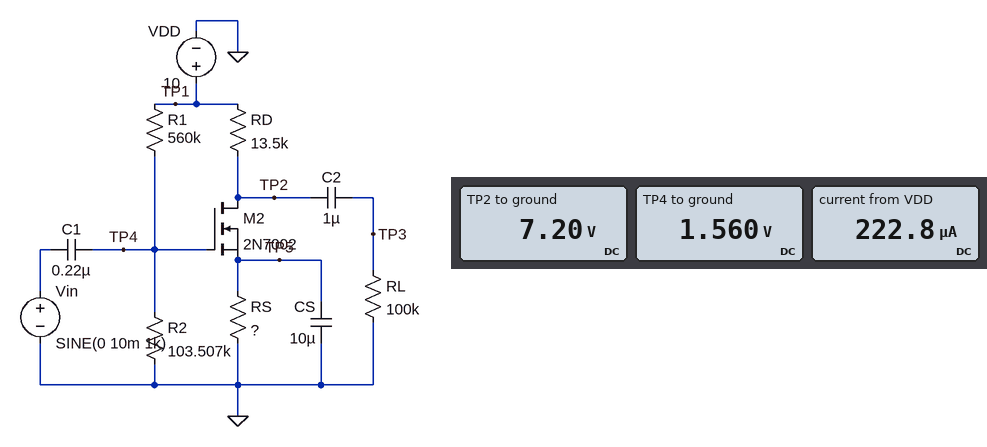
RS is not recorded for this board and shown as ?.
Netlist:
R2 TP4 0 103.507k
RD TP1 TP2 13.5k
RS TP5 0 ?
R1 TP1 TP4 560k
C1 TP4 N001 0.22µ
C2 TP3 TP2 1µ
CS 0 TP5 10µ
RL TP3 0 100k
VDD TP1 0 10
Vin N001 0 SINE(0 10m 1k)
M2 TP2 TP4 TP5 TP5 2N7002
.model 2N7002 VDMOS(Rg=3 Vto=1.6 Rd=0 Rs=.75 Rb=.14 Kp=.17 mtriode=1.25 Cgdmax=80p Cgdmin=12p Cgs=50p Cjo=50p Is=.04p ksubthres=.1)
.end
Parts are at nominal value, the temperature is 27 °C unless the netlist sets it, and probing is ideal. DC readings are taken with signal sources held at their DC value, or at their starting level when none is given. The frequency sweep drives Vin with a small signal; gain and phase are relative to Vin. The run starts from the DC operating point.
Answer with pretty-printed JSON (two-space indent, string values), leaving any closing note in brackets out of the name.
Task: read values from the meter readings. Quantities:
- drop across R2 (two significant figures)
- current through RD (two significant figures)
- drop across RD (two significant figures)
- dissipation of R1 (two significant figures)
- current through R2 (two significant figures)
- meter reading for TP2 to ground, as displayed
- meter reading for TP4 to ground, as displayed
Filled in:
{
  "drop across R2": "1.6 V",
  "current through RD": "210 µA",
  "drop across RD": "2.8 V",
  "dissipation of R1": "130 µW",
  "current through R2": "15 µA",
  "meter reading for TP2 to ground, as displayed": "7.20 V",
  "meter reading for TP4 to ground, as displayed": "1.560 V"
}
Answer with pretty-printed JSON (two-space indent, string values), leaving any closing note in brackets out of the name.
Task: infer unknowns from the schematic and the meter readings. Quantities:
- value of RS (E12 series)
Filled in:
{
  "value of RS": "22 Ω"
}
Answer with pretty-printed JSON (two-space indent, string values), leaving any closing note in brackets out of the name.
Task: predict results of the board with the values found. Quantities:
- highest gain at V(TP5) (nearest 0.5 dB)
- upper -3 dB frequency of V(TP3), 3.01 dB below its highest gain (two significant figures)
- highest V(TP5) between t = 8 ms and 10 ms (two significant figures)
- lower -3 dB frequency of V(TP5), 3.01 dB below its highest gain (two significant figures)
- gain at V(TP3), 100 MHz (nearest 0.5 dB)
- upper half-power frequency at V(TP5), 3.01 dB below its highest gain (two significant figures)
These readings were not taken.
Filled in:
{
  "highest gain at V(TP5)": "-23.5 dB",
  "upper -3 dB frequency of V(TP3), 3.01 dB below its highest gain": "410 kHz",
  "highest V(TP5) between t = 8 ms and 10 ms": "5.0 mV",
  "lower -3 dB frequency of V(TP5), 3.01 dB below its highest gain": "8.1 Hz",
  "gain at V(TP3), 100 MHz": "-5.5 dB",
  "upper half-power frequency at V(TP5), 3.01 dB below its highest gain": "790 Hz"
}
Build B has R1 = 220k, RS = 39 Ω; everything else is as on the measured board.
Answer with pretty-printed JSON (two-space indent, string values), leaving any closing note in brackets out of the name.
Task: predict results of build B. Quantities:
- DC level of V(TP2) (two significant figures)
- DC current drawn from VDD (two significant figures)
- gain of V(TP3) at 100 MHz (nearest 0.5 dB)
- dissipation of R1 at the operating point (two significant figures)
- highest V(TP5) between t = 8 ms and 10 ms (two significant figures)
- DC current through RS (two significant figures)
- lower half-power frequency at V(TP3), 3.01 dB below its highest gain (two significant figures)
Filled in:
{
  "DC level of V(TP2)": "32 mV",
  "DC current drawn from VDD": "770 µA",
  "gain of V(TP3) at 100 MHz": "-14.5 dB",
  "dissipation of R1 at the operating point": "210 µW",
  "highest V(TP5) between t = 8 ms and 10 ms": "29 mV",
  "DC current through RS": "740 µA",
  "lower half-power frequency at V(TP3), 3.01 dB below its highest gain": "160 MHz"
}
